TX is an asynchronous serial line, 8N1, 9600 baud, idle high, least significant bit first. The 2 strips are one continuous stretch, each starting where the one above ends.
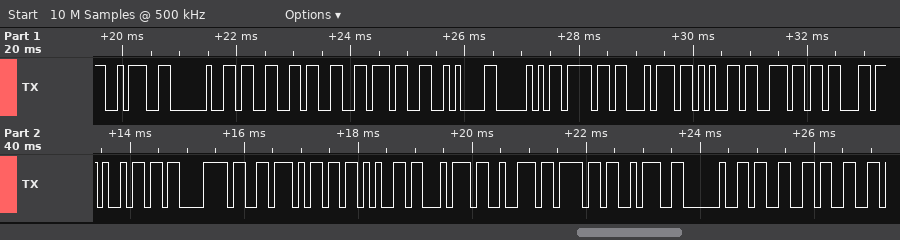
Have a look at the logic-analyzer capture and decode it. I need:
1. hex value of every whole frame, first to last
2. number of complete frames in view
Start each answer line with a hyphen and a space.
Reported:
- 3A 20 33 33 37 0A 50 6F 74 65 6E 63 69 C3 B3 6D 65 74 72 6F 3A 20 33 33
- 24
